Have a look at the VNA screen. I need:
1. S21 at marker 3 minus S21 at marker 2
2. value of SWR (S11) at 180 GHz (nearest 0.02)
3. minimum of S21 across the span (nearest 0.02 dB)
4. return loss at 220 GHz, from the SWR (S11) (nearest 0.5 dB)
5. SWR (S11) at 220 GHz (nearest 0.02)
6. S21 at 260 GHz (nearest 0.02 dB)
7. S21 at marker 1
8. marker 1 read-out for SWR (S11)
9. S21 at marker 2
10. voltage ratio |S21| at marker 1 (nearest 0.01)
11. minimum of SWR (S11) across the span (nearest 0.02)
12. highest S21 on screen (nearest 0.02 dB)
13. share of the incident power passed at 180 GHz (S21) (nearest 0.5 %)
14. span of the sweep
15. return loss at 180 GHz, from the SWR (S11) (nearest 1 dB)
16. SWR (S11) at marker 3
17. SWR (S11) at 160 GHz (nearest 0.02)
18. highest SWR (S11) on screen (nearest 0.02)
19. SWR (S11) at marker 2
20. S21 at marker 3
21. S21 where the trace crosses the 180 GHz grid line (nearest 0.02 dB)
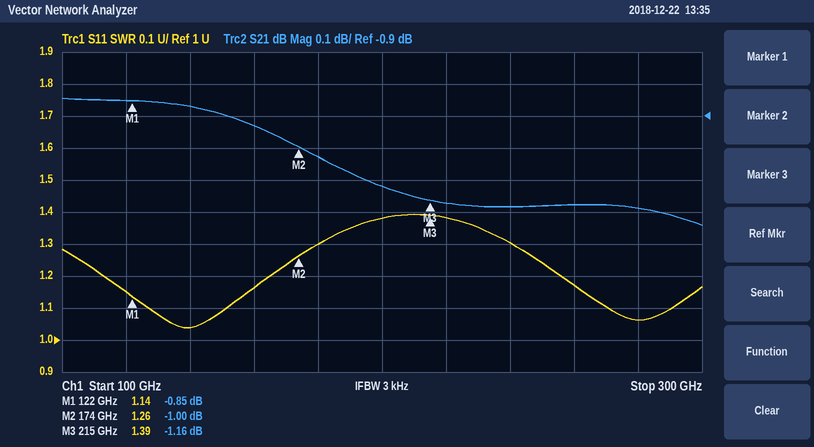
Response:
-0.16 dB
1.30
-1.24 dB
16.0 dB
1.38
-1.18 dB
-0.85 dB
1.14
-1.00 dB
0.91
1.04
-0.84 dB
79.0 %
200 GHz
18 dB
1.39
1.16
1.40
1.26
-1.16 dB
-1.02 dB
